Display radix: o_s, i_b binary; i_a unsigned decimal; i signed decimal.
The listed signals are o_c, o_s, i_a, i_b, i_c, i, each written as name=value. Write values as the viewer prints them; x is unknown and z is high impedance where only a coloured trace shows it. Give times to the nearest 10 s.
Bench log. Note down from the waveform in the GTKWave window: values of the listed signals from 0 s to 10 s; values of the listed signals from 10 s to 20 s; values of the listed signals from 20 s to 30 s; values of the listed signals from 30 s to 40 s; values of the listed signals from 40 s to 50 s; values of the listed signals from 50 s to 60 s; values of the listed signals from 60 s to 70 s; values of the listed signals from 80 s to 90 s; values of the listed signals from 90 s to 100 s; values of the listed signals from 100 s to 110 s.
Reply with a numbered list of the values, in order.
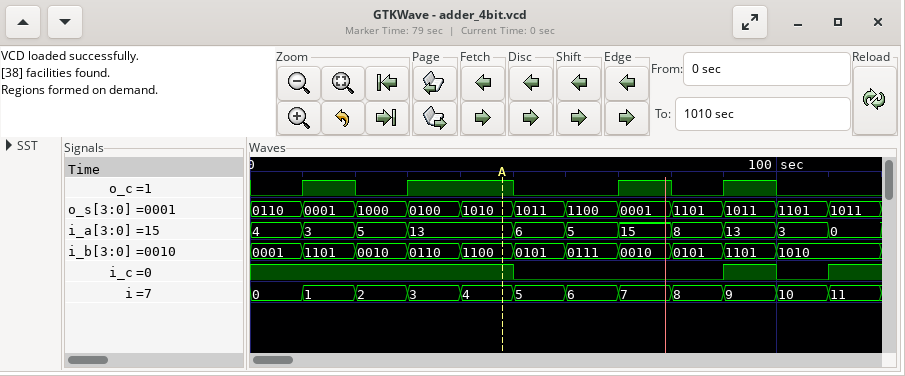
1. o_c=0, o_s=0110, i_a=4, i_b=0001, i_c=1, i=0
2. o_c=1, o_s=0001, i_a=3, i_b=1101, i_c=1, i=1
3. o_c=0, o_s=1000, i_a=5, i_b=0010, i_c=1, i=2
4. o_c=1, o_s=0100, i_a=13, i_b=0110, i_c=1, i=3
5. o_c=1, o_s=1010, i_a=13, i_b=1100, i_c=1, i=4
6. o_c=0, o_s=1011, i_a=6, i_b=0101, i_c=0, i=5
7. o_c=0, o_s=1100, i_a=5, i_b=0111, i_c=0, i=6
8. o_c=0, o_s=1101, i_a=8, i_b=0101, i_c=0, i=8
9. o_c=1, o_s=1011, i_a=13, i_b=1101, i_c=1, i=9
10. o_c=0, o_s=1101, i_a=3, i_b=1010, i_c=0, i=10
